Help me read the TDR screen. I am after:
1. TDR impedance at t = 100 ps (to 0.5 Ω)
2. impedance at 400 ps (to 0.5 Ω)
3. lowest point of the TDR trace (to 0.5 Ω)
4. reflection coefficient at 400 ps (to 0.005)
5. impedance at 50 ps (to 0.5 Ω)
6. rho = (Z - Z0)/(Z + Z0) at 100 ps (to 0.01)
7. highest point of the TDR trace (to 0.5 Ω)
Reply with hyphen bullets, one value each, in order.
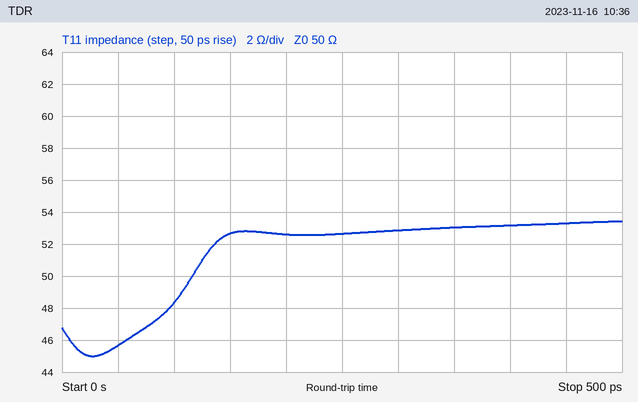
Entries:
- 48.5 Ω
- 53.0 Ω
- 45.0 Ω
- +0.030
- 45.5 Ω
- -0.02
- 53.5 Ω
